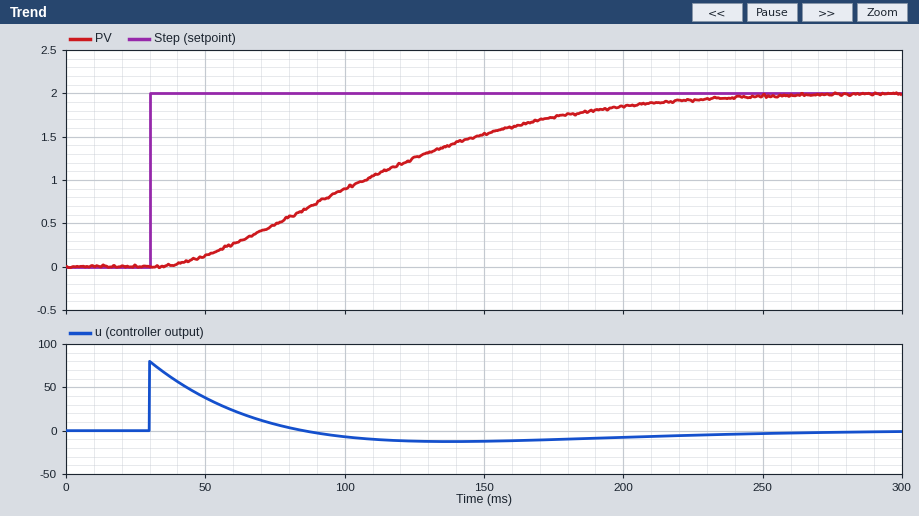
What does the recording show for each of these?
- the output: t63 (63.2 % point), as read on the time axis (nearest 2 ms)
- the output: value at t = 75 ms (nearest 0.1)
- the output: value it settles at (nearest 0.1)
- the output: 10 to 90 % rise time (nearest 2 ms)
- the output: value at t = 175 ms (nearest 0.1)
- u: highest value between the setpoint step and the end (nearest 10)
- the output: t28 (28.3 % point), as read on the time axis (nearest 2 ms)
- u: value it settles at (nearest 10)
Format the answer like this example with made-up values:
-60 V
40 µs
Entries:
126 ms
0.5
2.0
132 ms
1.7
80
80 ms
0
